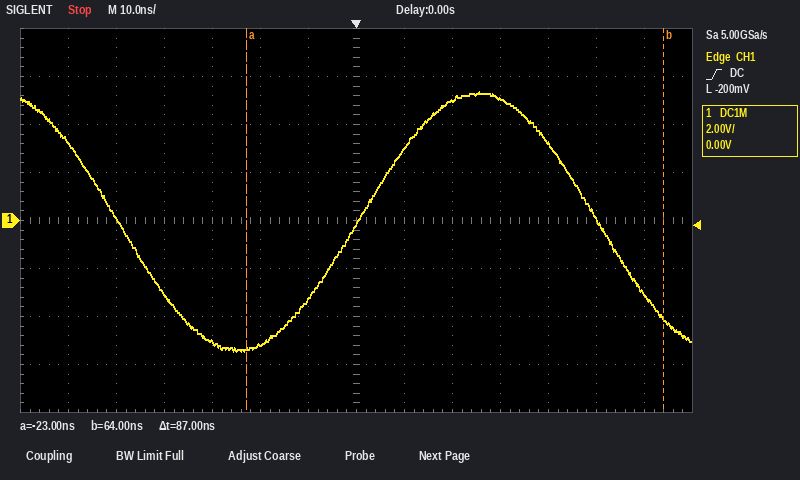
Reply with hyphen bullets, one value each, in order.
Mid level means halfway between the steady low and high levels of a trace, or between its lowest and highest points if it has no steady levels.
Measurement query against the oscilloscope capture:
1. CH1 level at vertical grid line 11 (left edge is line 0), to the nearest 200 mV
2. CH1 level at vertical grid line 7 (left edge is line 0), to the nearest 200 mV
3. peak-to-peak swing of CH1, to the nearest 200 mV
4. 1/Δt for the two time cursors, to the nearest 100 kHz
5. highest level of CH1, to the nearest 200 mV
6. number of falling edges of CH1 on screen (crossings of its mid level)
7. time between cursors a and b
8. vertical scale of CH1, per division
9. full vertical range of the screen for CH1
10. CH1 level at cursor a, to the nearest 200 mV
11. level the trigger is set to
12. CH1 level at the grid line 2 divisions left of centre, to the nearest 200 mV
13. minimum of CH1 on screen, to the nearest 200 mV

- 3.2 V
- -200 mV
- 10.8 V
- 11.5 MHz
- 5.4 V
- 2
- 87 ns
- 2 V
- 16 V
- -5.4 V
- -200 mV
- -5.2 V
- -5.4 V
